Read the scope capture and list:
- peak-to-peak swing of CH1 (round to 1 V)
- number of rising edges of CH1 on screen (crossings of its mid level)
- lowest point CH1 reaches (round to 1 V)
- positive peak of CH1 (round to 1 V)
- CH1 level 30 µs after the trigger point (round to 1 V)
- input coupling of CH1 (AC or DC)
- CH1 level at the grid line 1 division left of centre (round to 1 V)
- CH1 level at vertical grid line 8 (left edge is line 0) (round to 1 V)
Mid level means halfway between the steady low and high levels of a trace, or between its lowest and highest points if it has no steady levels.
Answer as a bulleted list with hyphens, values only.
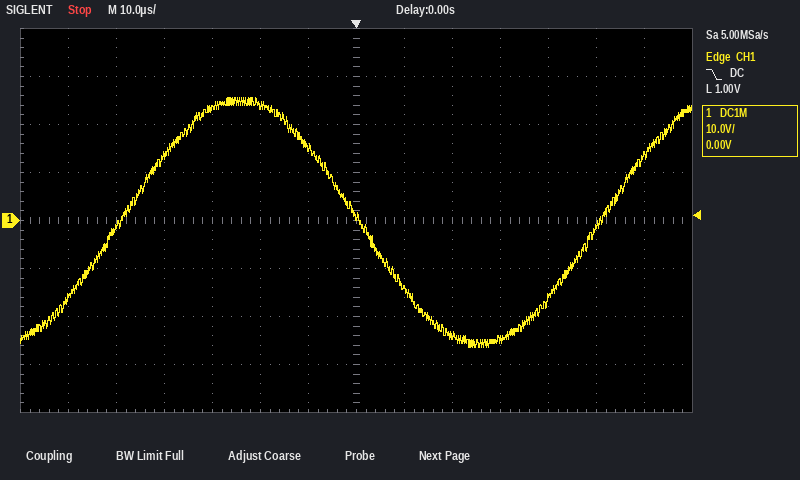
- 52 V
- 2
- -26 V
- 26 V
- -25 V
- DC
- 15 V
- -14 V
